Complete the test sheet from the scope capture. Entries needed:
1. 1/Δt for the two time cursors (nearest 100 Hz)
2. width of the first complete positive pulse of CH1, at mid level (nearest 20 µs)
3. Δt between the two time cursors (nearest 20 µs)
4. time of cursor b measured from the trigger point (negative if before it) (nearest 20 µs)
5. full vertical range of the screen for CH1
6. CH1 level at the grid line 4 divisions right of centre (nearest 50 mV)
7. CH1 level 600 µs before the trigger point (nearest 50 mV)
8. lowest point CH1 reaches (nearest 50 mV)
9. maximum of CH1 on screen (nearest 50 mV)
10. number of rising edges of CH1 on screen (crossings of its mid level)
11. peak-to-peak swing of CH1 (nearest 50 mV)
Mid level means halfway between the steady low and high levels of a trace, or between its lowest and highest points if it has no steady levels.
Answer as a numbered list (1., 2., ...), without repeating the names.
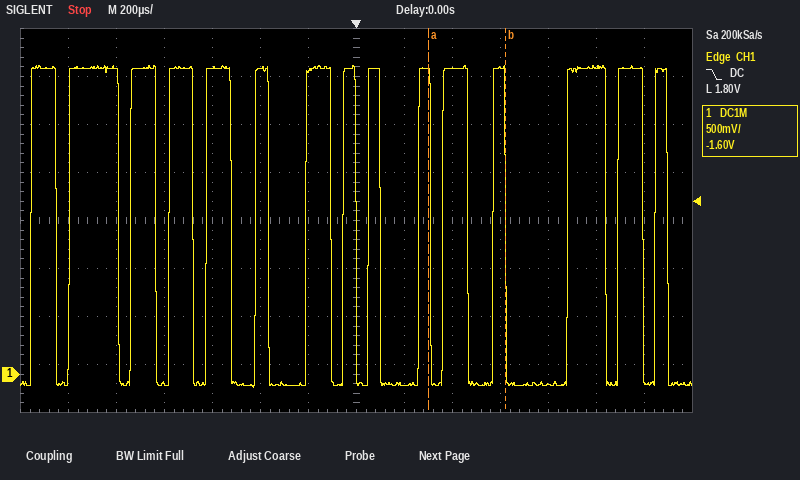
1. 3.1 kHz
2. 100 µs
3. 320 µs
4. +620 µs
5. 4 V
6. -100 mV
7. 3.20 V
8. -150 mV
9. 3.20 V
10. 15
11. 3.35 V
